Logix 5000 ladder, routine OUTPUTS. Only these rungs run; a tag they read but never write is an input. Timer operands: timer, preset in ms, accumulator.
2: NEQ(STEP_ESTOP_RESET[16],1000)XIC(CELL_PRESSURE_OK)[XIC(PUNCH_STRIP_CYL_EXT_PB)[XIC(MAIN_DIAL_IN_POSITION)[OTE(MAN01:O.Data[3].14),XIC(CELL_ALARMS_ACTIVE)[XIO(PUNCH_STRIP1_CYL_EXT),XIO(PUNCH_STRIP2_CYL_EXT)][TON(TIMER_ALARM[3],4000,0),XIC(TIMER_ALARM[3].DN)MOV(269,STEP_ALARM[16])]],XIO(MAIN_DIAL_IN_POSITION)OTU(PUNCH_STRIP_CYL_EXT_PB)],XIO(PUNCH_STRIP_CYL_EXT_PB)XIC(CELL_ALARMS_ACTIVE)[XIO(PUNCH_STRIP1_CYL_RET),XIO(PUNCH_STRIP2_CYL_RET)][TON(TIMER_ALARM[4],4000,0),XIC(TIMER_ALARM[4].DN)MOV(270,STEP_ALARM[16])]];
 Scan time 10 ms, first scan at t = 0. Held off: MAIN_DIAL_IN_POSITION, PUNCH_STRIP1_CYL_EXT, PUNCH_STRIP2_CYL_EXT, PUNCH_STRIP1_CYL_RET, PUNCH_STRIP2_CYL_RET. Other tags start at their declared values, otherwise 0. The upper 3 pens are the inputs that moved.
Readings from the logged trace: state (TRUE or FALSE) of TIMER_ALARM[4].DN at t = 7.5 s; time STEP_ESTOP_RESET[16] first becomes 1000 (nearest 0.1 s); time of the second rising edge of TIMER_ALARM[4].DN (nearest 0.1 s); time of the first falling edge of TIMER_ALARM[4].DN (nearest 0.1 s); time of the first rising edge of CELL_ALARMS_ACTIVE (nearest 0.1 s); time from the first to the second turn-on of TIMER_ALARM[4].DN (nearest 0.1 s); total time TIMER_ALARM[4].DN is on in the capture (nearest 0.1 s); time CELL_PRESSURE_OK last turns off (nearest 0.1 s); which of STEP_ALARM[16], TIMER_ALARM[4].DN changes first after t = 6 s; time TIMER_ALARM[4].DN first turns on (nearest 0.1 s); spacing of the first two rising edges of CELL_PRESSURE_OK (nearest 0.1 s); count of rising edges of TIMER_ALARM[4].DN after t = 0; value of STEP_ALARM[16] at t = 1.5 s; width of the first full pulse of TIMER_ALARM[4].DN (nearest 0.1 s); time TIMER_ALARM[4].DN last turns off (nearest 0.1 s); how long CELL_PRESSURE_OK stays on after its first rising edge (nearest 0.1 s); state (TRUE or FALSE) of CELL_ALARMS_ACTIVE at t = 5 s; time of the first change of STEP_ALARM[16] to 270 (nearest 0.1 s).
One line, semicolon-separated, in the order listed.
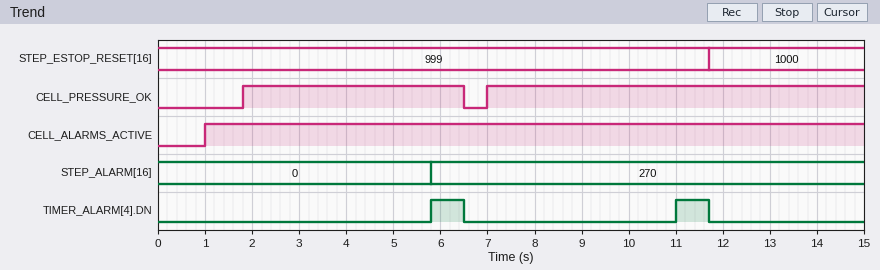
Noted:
FALSE; 11.7 s; 11.0 s; 6.5 s; 1.0 s; 5.2 s; 1.4 s; 6.5 s; TIMER_ALARM[4].DN; 5.8 s; 5.2 s; 2; 0; 0.7 s; 11.7 s; 4.7 s; TRUE; 5.8 s
